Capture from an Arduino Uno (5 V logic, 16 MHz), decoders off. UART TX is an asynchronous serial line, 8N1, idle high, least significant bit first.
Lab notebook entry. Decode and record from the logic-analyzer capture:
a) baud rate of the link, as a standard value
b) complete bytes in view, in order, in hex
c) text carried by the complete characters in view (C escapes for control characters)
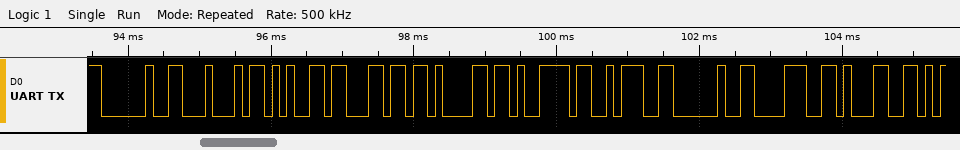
9600 baud
0x20 0x44 0x65 0x6C 0x61 0x79 0x3A 0x20 0x38 0x31
" Delay: 81"
